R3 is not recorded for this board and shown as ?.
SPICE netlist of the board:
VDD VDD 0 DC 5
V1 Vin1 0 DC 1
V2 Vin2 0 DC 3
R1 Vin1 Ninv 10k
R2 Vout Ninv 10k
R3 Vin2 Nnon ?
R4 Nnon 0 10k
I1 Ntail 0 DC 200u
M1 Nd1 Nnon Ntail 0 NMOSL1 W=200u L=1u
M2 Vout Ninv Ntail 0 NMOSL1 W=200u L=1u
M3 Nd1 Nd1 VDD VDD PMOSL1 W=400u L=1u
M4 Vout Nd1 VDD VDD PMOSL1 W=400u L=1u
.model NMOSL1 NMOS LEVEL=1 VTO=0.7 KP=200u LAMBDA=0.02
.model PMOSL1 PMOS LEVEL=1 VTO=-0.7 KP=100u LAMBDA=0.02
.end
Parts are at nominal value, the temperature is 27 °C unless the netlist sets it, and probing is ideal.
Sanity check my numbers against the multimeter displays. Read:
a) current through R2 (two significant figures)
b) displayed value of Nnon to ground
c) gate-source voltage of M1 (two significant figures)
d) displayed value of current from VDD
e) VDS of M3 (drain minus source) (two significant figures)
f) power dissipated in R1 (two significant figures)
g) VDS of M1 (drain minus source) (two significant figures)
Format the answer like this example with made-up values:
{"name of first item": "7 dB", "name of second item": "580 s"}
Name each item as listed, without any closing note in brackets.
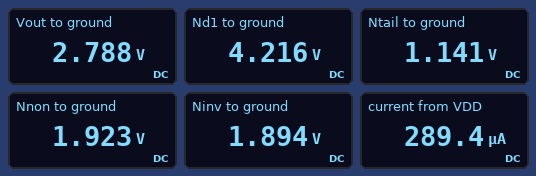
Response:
{"current through R2": "89 µA", "displayed value of Nnon to ground": "1.923 V", "gate-source voltage of M1": "780 mV", "displayed value of current from VDD": "289.4 µA", "VDS of M3 (drain minus source)": "-780 mV", "power dissipated in R1": "80 µW", "VDS of M1 (drain minus source)": "3.1 V"}
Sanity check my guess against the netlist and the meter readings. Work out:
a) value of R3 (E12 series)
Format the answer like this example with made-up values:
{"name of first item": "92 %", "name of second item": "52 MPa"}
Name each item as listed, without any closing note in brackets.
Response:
{"value of R3": "5.6 kΩ"}
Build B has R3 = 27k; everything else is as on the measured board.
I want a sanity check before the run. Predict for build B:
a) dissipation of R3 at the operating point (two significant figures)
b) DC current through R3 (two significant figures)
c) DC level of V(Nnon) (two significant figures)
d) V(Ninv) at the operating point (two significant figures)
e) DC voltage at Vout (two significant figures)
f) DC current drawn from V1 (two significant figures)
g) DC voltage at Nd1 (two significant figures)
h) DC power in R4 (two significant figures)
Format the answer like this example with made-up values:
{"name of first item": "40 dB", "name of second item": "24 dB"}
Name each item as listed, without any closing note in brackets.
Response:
{"dissipation of R3 at the operating point": "180 µW", "DC current through R3": "81 µA", "DC level of V(Nnon)": "810 mV", "V(Ninv) at the operating point": "820 mV", "DC voltage at Vout": "640 mV", "DC current drawn from V1": "18 µA", "DC voltage at Nd1": "4.2 V", "DC power in R4": "66 µW"}
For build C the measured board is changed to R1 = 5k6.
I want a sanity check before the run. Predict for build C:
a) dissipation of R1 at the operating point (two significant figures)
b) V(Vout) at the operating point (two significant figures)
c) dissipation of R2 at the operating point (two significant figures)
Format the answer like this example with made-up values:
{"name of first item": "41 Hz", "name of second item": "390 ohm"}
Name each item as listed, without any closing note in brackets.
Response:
{"dissipation of R1 at the operating point": "130 µW", "V(Vout) at the operating point": "3.4 V", "dissipation of R2 at the operating point": "240 µW"}
